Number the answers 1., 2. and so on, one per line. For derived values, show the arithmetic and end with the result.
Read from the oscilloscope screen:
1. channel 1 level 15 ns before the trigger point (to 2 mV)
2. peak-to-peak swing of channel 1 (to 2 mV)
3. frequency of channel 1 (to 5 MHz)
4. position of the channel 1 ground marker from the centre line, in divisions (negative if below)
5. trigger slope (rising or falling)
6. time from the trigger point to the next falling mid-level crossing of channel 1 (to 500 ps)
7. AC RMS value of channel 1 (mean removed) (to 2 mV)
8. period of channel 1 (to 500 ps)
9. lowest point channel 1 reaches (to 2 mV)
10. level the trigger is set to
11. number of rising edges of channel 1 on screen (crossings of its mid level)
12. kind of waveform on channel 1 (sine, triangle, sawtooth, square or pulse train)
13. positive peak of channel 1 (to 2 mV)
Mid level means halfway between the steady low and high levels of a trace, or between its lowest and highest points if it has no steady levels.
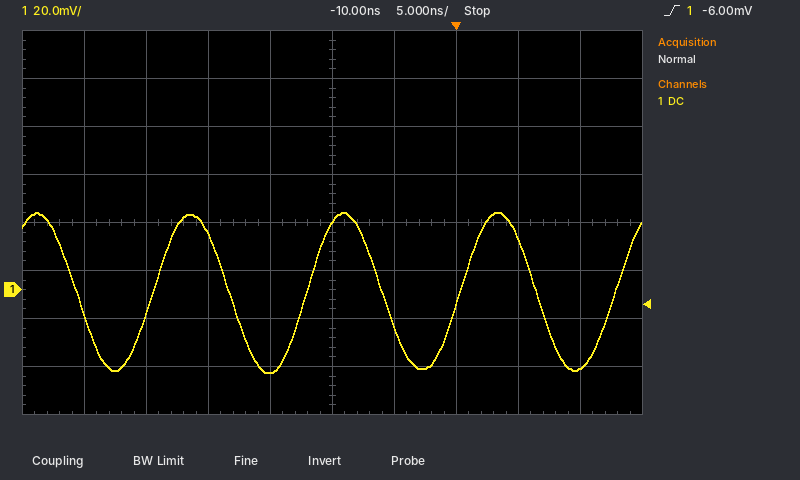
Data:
1. -34 mV
2. 32 mV − (-34 mV) = 66 mV
3. 1 / 12.5 ns ≈ 80 MHz
4. -1.4 div
5. rising
6. 6.5 ns
7. 66 mV / (2√2) ≈ 23.3 mV, so 24 mV to the nearest 2 mV
8. 12.5 ns
9. -34 mV
10. -6.00 mV
11. 4
12. sine
13. 32 mV
